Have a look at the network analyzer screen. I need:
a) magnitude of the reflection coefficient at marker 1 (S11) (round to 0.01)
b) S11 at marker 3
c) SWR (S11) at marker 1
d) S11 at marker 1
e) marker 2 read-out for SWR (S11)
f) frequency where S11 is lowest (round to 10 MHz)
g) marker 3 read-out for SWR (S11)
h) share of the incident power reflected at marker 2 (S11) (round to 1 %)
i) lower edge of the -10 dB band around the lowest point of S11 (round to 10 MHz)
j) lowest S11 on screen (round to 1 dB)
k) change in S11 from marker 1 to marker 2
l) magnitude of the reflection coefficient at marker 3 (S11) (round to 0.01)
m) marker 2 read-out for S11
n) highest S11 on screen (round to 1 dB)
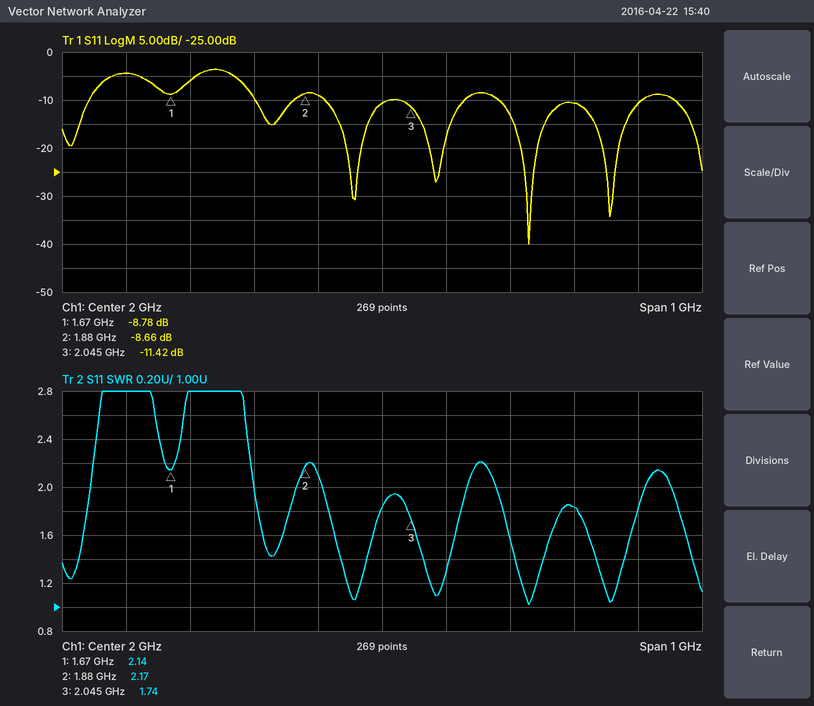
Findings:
0.36
-11.42 dB
2.14
-8.78 dB
2.17
2.23 GHz
1.74
14 %
2.18 GHz
-40 dB
0.12 dB
0.27
-8.66 dB
-4 dB
